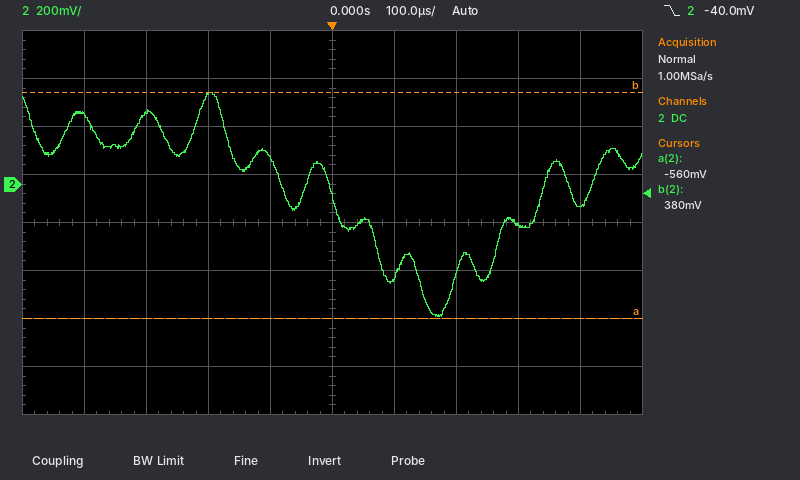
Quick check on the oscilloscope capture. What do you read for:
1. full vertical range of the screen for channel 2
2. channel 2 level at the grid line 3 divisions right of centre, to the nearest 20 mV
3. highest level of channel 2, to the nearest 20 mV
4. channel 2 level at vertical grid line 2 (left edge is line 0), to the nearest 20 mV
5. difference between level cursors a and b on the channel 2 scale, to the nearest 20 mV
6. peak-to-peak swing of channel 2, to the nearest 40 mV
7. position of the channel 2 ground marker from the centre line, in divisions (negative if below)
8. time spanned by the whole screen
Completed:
1.6 V
-180 mV
380 mV
300 mV
940 mV
920 mV
+0.8 div
1 ms
